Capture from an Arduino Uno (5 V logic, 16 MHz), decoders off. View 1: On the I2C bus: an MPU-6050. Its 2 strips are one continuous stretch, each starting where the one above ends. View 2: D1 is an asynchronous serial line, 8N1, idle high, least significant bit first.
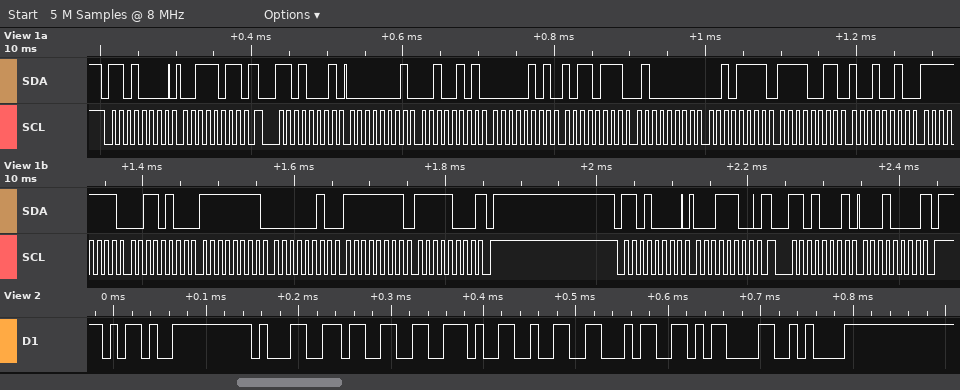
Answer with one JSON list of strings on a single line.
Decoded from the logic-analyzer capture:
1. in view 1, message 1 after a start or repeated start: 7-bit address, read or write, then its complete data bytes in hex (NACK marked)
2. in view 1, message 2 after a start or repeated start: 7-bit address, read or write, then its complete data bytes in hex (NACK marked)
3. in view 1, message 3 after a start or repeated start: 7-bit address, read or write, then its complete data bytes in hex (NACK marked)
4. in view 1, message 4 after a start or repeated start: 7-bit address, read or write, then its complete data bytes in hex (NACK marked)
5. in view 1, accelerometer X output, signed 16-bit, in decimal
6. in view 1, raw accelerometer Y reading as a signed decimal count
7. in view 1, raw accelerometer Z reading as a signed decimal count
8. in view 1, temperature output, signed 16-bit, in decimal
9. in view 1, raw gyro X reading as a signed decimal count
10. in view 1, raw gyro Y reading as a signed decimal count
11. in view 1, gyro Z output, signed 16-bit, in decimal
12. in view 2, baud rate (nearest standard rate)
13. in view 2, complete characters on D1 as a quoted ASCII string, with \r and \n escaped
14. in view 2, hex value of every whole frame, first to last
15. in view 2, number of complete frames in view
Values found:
["0x68 write: 3B", "0x68 read: 01 25 05 B7 40 2F F3 92 FF 34 FF 02 FF F8 NACK", "0x68 write: 1C", "0x68 read: 10 NACK", "293", "1463", "16431", "-3182", "-204", "-254", "-8", "115200 baud", "\"-13.24\\r\\n\"", "2D 31 33 2E 32 34 0D 0A", "8"]
